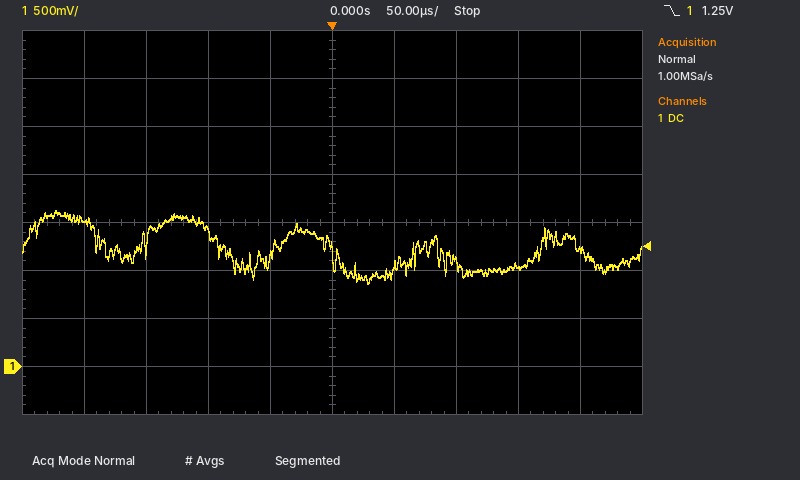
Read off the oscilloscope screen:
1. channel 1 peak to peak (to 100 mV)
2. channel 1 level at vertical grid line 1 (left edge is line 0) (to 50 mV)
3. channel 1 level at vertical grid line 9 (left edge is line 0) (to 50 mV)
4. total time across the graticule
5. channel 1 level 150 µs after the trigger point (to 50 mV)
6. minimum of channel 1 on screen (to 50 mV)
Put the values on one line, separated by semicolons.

800 mV; 1.50 V; 1.20 V; 500 µs; 1.05 V; 850 mV
